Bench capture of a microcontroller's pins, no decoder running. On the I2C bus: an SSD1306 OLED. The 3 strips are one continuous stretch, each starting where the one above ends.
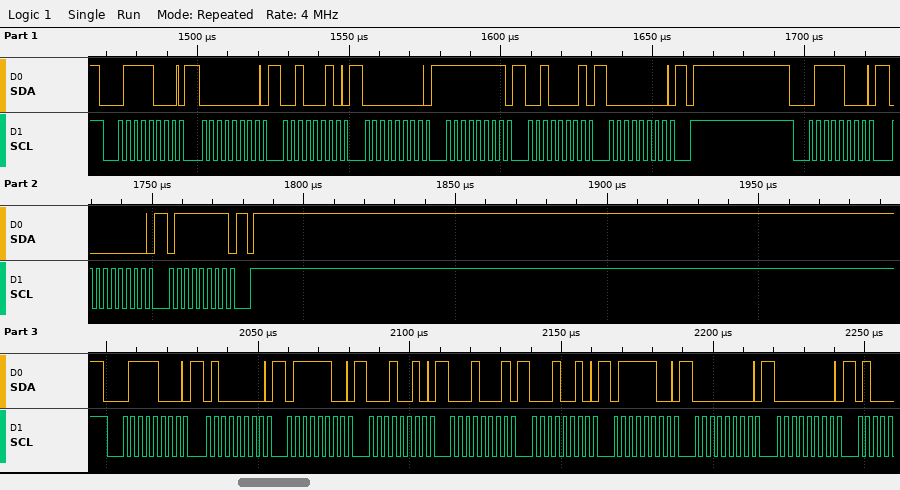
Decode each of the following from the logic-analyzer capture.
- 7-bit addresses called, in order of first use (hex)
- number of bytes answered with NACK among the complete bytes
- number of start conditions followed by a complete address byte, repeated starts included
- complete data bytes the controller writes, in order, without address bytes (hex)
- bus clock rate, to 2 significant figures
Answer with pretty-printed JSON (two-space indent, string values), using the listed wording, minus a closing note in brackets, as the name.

{
  "7-bit addresses called, in order of first use": "0x3C",
  "number of bytes answered with NACK among the complete bytes": "0",
  "number of start conditions followed by a complete address byte, repeated starts included": "3",
  "complete data bytes the controller writes, in order, without address bytes": "00 22 00 FF 21 00 00 7F 40 7C 12 11 12 7C 00 00",
  "bus clock rate, to 2 significant figures": "400 kHz"
}
